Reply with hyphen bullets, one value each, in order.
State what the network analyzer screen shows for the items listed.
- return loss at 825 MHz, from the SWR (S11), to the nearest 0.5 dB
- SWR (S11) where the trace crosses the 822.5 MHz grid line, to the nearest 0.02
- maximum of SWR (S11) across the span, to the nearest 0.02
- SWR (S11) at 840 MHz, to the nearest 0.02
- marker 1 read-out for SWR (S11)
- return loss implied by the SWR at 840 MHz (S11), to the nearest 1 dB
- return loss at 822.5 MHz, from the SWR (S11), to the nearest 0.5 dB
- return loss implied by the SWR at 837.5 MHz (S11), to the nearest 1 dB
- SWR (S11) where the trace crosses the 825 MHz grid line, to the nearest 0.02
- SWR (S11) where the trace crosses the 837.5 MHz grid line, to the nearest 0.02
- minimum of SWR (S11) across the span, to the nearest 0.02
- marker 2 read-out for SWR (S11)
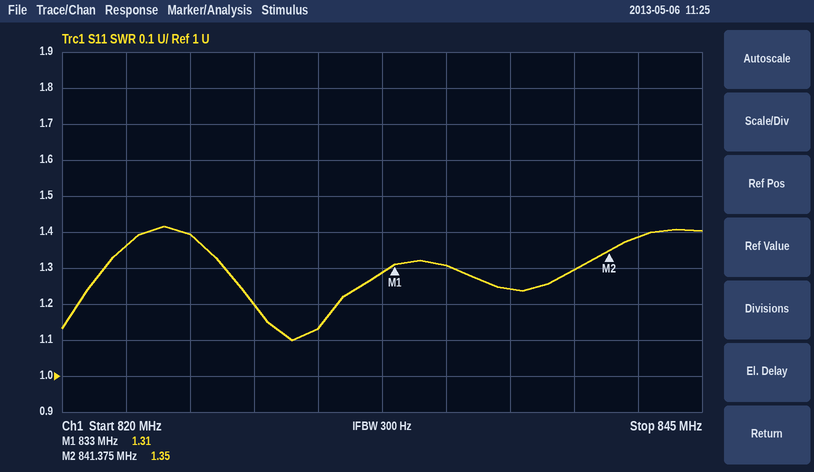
- 15.5 dB
- 1.36
- 1.42
- 1.30
- 1.31
- 18 dB
- 16.5 dB
- 19 dB
- 1.40
- 1.24
- 1.10
- 1.35
